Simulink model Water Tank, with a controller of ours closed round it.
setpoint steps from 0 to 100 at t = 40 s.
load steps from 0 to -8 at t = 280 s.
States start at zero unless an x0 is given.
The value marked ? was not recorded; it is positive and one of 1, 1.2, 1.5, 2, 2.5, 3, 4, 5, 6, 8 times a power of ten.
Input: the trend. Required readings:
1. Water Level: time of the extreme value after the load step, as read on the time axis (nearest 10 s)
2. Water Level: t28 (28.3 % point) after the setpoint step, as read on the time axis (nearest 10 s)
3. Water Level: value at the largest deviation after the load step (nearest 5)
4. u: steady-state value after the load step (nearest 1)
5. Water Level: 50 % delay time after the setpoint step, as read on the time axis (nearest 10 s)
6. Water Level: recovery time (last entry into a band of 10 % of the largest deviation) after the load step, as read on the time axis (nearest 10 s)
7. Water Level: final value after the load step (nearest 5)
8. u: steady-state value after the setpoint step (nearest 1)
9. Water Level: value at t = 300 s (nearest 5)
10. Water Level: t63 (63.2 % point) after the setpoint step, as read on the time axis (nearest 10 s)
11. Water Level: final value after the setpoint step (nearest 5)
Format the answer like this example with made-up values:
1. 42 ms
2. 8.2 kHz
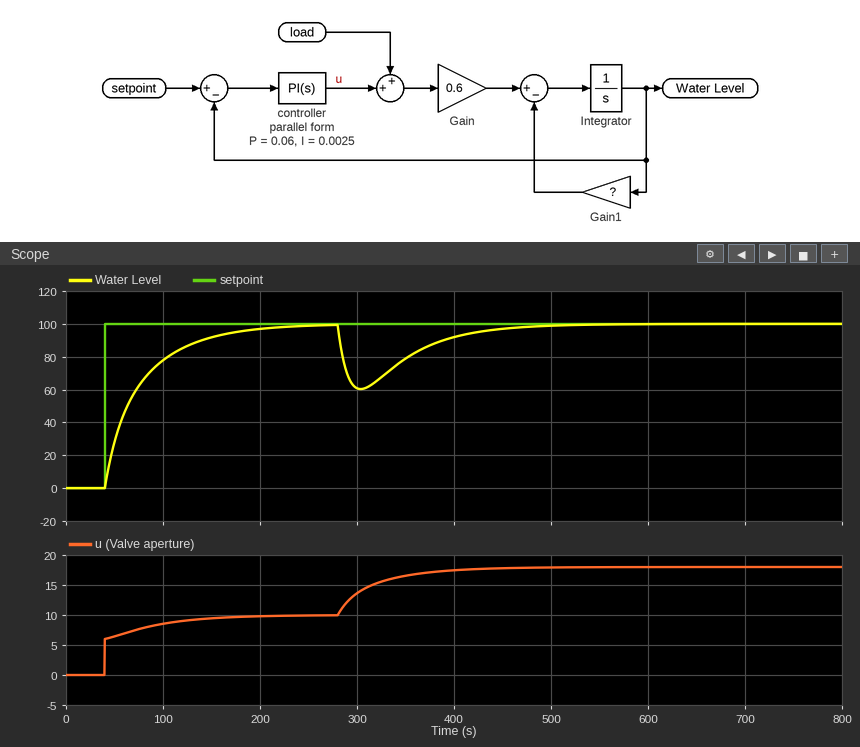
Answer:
1. 300 s
2. 50 s
3. 60
4. 18
5. 60 s
6. 440 s
7. 100
8. 10
9. 60
10. 80 s
11. 100
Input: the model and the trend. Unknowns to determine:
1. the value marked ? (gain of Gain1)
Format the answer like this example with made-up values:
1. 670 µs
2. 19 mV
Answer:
1. 0.06
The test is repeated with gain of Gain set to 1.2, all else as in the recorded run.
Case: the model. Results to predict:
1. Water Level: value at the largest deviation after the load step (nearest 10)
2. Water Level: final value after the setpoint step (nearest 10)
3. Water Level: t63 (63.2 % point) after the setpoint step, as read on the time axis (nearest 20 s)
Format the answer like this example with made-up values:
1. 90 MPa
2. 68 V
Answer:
1. 40
2. 100
3. 60 s
